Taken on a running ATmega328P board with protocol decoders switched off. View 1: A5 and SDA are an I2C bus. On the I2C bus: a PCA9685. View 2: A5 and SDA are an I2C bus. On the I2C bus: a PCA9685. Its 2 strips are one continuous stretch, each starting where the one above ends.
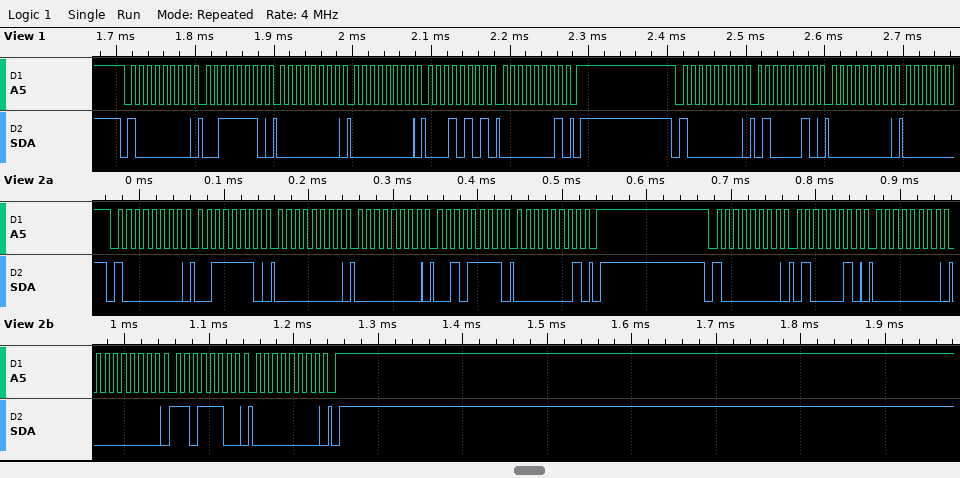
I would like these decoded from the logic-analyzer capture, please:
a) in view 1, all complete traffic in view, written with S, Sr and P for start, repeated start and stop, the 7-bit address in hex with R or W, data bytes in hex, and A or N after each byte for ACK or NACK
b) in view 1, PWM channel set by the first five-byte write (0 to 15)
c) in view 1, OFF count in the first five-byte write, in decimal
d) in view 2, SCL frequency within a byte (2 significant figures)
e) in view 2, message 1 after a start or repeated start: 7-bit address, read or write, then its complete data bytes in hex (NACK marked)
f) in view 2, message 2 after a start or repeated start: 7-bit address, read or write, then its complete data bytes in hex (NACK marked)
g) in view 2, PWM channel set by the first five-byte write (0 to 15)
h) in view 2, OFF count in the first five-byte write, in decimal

S 40W A 3E A 00 A 00 A 15 A 01 A P S 40W A 42 A 00 A
14
277
100 kHz
0x40 write: 3E 00 00 2F 01
0x40 write: 42 00 00 DC 00
14
303
